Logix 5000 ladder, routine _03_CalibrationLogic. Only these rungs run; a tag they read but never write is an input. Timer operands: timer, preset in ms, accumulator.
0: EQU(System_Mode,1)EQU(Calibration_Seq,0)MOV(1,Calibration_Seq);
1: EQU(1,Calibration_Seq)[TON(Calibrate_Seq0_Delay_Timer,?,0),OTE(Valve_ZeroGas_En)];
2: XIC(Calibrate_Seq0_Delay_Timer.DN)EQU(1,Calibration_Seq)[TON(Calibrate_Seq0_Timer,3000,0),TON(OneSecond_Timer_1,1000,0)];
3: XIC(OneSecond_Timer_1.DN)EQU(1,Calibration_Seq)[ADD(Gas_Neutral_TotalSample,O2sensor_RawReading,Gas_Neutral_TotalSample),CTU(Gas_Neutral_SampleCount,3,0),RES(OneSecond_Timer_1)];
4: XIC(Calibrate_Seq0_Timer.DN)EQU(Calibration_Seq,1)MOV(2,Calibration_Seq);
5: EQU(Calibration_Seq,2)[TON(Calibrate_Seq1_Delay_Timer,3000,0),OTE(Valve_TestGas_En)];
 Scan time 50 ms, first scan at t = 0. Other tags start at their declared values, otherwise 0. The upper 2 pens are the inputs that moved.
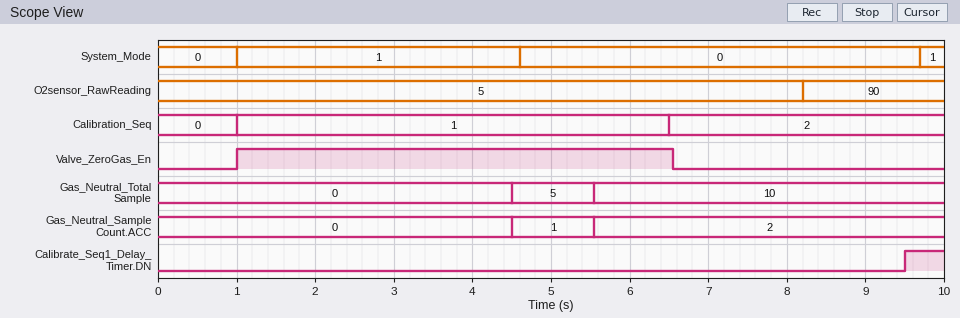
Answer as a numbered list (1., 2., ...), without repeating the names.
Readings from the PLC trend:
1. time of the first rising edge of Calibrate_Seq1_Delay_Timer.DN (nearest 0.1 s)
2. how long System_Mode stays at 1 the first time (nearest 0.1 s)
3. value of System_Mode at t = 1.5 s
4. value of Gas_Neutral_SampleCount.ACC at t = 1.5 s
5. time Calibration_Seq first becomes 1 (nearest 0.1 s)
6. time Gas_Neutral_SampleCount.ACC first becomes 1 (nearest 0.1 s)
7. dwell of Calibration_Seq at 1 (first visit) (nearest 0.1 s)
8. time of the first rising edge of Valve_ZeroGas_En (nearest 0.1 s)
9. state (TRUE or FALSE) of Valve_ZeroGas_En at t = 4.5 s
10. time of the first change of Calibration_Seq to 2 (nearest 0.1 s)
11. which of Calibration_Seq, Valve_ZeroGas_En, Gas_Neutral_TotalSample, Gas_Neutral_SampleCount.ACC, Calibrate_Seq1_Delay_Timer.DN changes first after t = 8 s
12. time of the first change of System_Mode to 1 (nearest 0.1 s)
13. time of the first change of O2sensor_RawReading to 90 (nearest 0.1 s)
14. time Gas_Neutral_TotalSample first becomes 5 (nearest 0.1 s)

1. 9.5 s
2. 3.6 s
3. 1
4. 0
5. 1.0 s
6. 4.5 s
7. 5.5 s
8. 1.0 s
9. TRUE
10. 6.5 s
11. Calibrate_Seq1_Delay_Timer.DN
12. 1.0 s
13. 8.2 s
14. 4.5 s
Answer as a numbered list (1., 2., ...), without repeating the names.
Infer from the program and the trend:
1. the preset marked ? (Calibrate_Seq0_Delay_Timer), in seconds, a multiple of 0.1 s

1. 2.5 s
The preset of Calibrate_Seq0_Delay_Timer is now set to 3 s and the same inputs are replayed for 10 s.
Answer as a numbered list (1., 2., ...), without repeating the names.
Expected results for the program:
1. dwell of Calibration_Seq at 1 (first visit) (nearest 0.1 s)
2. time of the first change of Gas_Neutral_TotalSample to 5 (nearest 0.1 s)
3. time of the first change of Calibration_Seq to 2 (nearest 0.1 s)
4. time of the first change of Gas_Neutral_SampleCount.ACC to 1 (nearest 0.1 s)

1. 6.0 s
2. 5.0 s
3. 7.0 s
4. 5.0 s
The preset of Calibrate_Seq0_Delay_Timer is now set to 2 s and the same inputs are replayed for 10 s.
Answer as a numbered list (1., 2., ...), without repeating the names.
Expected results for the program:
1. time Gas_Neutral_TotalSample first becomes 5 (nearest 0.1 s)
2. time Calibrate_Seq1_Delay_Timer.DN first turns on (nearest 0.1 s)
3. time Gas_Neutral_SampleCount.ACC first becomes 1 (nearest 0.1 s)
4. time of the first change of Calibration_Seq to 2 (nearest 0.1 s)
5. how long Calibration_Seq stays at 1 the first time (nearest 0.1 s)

1. 4.0 s
2. 9.0 s
3. 4.0 s
4. 6.0 s
5. 5.0 s
